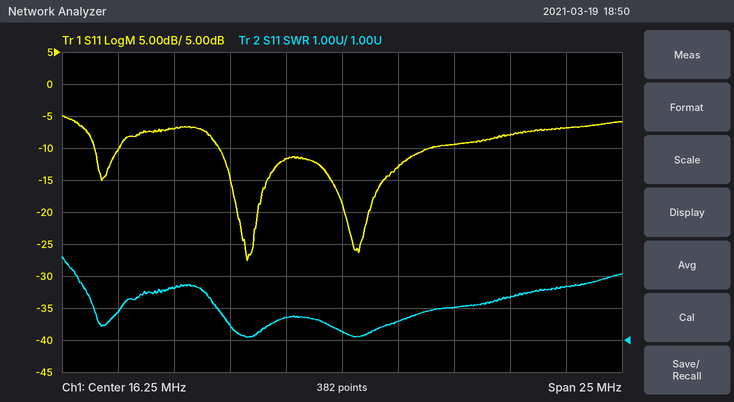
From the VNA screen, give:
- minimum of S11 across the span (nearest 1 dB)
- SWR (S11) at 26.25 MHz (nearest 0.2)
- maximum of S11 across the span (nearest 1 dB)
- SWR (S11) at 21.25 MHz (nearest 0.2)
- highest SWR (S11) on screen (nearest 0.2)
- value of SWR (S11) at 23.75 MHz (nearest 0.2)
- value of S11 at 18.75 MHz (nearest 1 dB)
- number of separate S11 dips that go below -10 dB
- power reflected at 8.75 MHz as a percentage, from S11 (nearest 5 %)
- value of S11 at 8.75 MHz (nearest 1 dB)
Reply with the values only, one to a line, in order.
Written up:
-28 dB
2.6
-5 dB
2.0
3.6
2.4
-13 dB
3
20 %
-7 dB
